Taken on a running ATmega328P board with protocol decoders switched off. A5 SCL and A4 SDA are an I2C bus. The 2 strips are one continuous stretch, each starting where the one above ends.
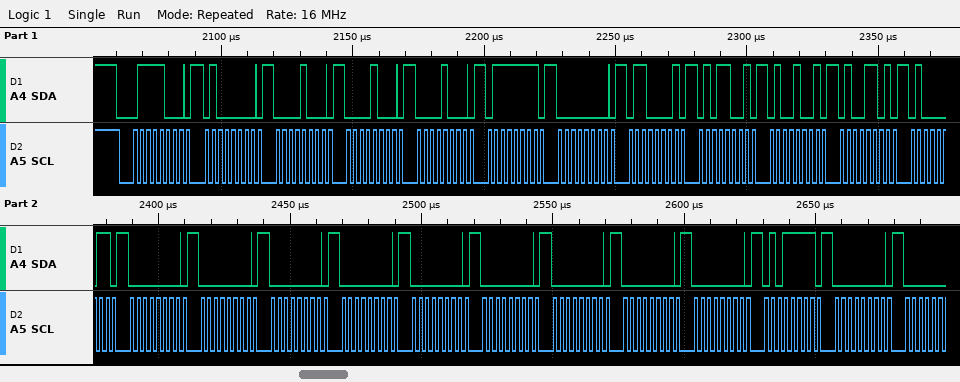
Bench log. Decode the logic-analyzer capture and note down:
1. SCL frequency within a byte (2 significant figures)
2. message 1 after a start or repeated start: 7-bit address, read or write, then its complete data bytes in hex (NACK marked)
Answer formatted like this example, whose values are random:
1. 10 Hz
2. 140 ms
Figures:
1. 400 kHz
2. 0x3C write: 40 08 08 08 7F 00 61 59 49 4D 43 00 00 00 00 00 00 00 00 00 5F 00
